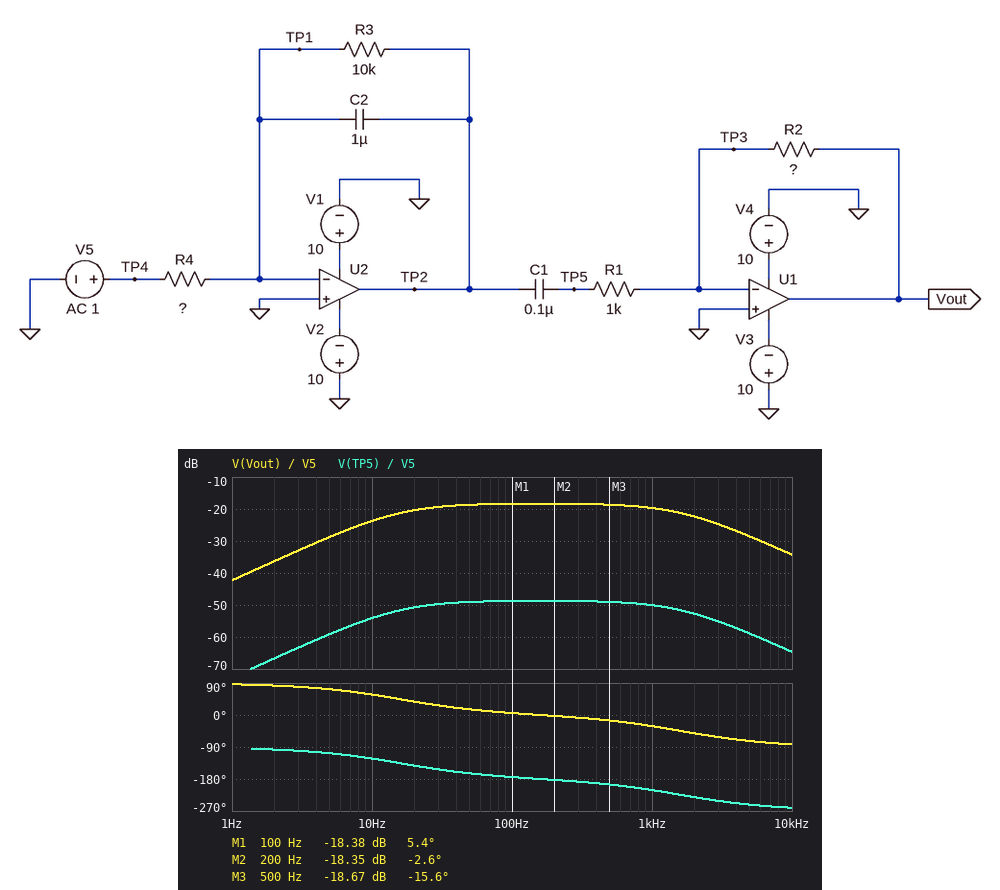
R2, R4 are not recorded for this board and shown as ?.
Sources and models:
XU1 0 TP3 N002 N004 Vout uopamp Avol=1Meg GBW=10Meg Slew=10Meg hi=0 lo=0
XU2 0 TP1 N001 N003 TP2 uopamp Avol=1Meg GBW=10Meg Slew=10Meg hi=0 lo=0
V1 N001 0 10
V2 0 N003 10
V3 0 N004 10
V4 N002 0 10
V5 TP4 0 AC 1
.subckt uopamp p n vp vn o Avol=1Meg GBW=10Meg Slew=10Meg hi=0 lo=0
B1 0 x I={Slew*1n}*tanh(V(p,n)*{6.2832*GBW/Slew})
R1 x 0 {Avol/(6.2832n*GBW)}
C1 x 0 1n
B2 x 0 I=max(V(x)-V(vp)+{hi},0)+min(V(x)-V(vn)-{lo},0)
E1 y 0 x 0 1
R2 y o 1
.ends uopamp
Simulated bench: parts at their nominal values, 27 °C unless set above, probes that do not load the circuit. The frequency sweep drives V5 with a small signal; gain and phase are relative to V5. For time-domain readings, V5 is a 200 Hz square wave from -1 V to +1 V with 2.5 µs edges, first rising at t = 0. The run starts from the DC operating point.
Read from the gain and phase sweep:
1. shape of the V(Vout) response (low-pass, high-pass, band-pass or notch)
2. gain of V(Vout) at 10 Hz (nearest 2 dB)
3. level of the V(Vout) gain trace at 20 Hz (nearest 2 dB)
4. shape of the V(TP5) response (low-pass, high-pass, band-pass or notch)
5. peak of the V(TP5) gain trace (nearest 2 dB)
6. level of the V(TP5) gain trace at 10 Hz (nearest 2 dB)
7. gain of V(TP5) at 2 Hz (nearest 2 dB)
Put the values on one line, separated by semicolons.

band-pass; -24 dB; -20 dB; band-pass; -48 dB; -54 dB; -66 dB
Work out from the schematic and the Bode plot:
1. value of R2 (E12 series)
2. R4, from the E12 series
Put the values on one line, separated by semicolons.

33 kΩ; 27 kΩ
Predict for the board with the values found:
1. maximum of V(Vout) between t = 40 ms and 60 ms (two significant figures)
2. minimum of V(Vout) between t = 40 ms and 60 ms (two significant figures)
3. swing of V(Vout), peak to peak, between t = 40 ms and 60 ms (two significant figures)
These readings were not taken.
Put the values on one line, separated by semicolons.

130 mV; -130 mV; 260 mV
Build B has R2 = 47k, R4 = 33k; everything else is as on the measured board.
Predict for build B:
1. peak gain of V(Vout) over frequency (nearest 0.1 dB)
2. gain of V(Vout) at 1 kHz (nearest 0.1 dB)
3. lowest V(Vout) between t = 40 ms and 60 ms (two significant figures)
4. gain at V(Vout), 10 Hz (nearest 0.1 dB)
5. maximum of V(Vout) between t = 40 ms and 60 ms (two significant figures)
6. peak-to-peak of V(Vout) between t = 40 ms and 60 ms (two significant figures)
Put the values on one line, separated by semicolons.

-17.0 dB; -18.4 dB; -150 mV; -22.4 dB; 150 mV; 310 mV
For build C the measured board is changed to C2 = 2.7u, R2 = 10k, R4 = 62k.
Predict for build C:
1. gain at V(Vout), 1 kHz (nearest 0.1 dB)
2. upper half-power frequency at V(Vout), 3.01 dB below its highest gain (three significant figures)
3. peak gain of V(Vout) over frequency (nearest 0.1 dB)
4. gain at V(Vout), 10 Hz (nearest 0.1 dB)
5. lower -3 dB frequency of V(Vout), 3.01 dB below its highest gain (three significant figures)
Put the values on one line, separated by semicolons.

-45.9 dB; 1.61 kHz; -44.5 dB; -45.8 dB; 5.85 Hz
